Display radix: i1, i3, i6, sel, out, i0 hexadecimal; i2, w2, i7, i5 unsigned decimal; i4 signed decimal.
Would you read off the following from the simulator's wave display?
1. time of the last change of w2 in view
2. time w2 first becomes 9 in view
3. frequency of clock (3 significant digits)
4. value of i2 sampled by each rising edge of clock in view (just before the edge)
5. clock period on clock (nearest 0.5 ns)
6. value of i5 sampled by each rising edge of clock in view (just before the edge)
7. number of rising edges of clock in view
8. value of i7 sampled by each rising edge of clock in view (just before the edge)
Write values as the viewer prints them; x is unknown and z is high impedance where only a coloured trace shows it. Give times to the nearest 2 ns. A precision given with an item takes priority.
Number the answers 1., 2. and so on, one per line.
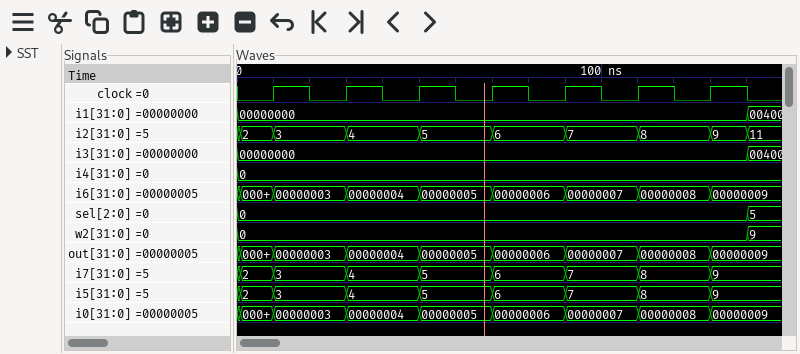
1. 140 ns
2. 140 ns
3. 50.0 MHz
4. 2, 3, 4, 5, 6, 7, 8
5. 20 ns
6. 2, 3, 4, 5, 6, 7, 8
7. 7
8. 2, 3, 4, 5, 6, 7, 8
